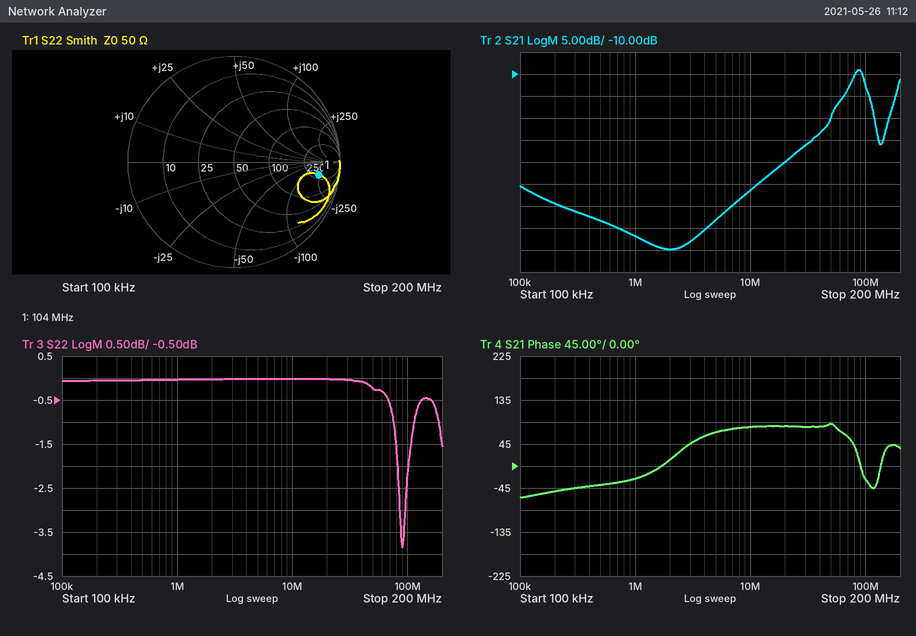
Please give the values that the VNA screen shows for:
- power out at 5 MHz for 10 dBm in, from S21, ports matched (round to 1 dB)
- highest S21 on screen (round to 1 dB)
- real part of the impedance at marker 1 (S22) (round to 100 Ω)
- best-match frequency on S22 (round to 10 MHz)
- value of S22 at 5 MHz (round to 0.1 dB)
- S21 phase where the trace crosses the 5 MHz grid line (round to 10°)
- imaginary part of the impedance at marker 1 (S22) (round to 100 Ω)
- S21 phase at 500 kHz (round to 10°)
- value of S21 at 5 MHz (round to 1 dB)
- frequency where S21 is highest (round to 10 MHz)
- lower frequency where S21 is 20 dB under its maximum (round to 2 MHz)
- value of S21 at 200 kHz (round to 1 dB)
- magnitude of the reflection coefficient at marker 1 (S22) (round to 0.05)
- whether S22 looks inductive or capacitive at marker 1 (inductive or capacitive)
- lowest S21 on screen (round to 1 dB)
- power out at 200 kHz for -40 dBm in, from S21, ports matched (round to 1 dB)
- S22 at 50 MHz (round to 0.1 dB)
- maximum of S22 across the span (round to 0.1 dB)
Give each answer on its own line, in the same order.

-33 dBm
-9 dB
300 Ω
90 MHz
0.0 dB
70°
-200 Ω
-40°
-43 dB
90 MHz
22 MHz
-39 dB
0.80
capacitive
-50 dB
-79 dBm
-0.2 dB
0.0 dB
